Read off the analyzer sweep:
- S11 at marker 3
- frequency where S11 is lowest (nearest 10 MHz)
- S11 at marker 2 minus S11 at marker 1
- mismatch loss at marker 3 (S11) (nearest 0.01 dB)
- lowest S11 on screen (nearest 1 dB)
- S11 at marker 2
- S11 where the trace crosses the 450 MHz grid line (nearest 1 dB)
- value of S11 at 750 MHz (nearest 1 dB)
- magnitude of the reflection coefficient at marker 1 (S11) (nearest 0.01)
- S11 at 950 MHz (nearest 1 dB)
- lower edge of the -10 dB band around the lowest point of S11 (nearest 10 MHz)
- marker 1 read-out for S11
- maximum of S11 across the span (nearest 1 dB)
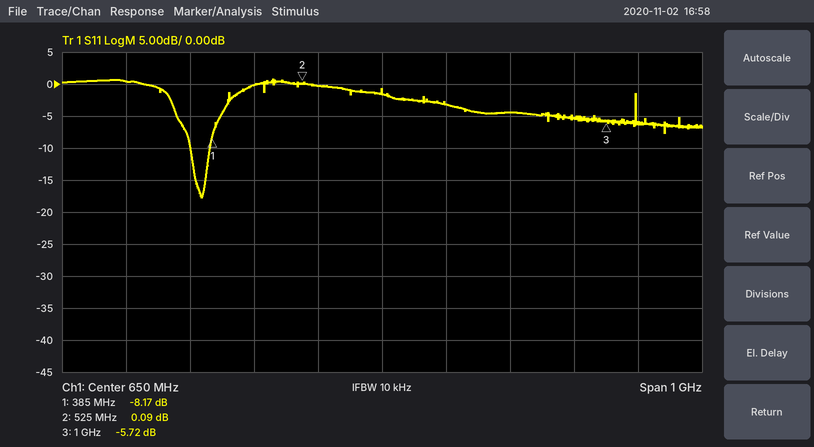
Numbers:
-5.72 dB
370 MHz
8.26 dB
1.35 dB
-18 dB
0.09 dB
0 dB
-3 dB
0.39
-5 dB
350 MHz
-8.17 dB
1 dB
